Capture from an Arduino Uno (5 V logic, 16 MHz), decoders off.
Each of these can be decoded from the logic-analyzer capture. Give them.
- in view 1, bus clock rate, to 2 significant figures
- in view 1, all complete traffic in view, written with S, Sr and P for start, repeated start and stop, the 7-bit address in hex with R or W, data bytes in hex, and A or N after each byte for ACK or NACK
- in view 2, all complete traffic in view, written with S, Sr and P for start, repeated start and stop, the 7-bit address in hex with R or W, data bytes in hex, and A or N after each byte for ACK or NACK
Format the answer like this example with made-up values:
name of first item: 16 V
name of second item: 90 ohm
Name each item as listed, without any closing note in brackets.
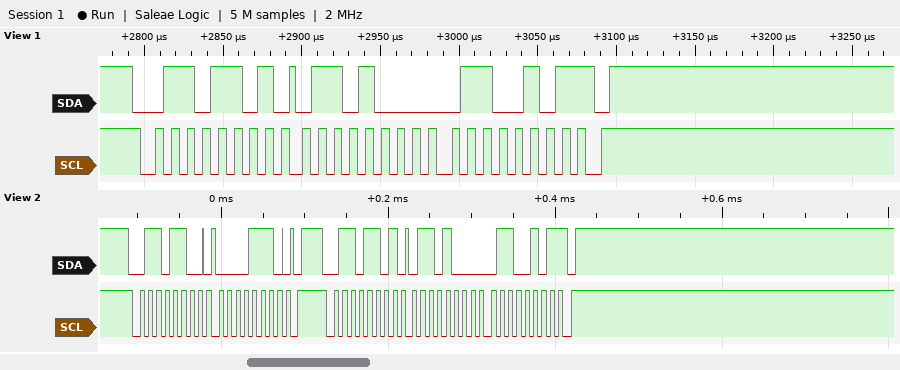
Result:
in view 1, bus clock rate, to 2 significant figures: 100 kHz
in view 1, all complete traffic in view, written with S, Sr and P for start, repeated start and stop, the 7-bit address in hex with R or W, data bytes in hex, and A or N after each byte for ACK or NACK: S 36R A 68 A 65 N P
in view 2, all complete traffic in view, written with S, Sr and P for start, repeated start and stop, the 7-bit address in hex with R or W, data bytes in hex, and A or N after each byte for ACK or NACK: S 36W A 0E A P S 36R A 68 A 65 N P
